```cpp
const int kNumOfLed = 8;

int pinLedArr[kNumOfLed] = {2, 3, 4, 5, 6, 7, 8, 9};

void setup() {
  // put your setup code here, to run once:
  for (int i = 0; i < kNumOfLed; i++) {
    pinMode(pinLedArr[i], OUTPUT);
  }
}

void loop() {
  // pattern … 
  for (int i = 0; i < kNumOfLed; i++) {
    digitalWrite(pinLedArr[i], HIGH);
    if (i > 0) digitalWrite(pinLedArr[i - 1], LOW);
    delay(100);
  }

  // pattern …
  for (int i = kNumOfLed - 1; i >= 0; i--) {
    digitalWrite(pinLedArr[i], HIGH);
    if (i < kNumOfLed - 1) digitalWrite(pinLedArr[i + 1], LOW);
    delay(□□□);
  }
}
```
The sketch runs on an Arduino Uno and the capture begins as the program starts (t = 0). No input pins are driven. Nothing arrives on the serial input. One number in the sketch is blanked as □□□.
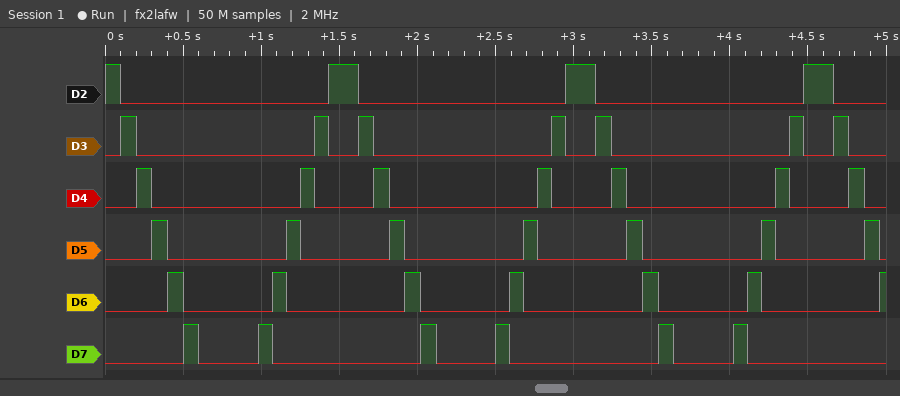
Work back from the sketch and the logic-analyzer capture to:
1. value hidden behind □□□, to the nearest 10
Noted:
90
